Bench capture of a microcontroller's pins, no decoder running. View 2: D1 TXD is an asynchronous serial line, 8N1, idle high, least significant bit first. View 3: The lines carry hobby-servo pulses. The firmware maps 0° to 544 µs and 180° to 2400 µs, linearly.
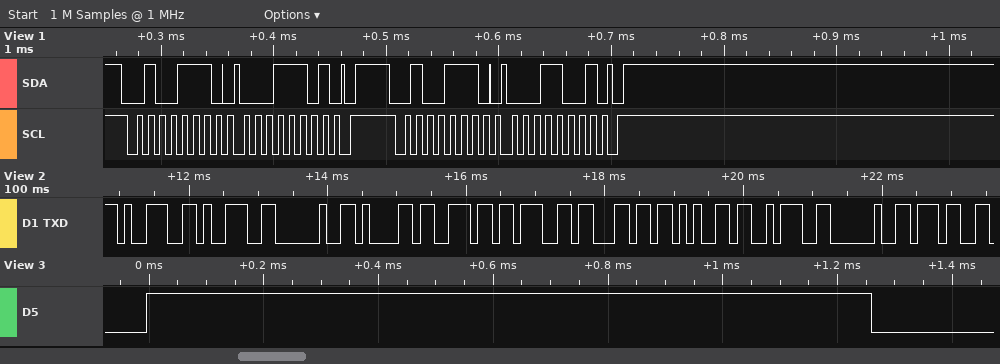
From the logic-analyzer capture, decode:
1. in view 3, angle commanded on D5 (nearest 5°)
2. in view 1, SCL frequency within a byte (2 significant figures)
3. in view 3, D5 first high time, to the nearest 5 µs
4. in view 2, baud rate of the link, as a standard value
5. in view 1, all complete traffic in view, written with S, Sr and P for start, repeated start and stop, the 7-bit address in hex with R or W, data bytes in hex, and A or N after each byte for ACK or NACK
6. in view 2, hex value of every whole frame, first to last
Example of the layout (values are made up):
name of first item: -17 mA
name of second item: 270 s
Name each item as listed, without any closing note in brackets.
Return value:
in view 3, angle commanded on D5: 70°
in view 1, SCL frequency within a byte: 100 kHz
in view 3, D5 first high time, to the nearest 5 µs: 1265 µs
in view 2, baud rate of the link, as a standard value: 9600 baud
in view 1, all complete traffic in view, written with S, Sr and P for start, repeated start and stop, the 7-bit address in hex with R or W, data bytes in hex, and A or N after each byte for ACK or NACK: S 27W A 1D A P S 27W A 19 A P
in view 2, hex value of every whole frame, first to last: 39 39 20 61 6E 67 6C 65 3A 20 37
